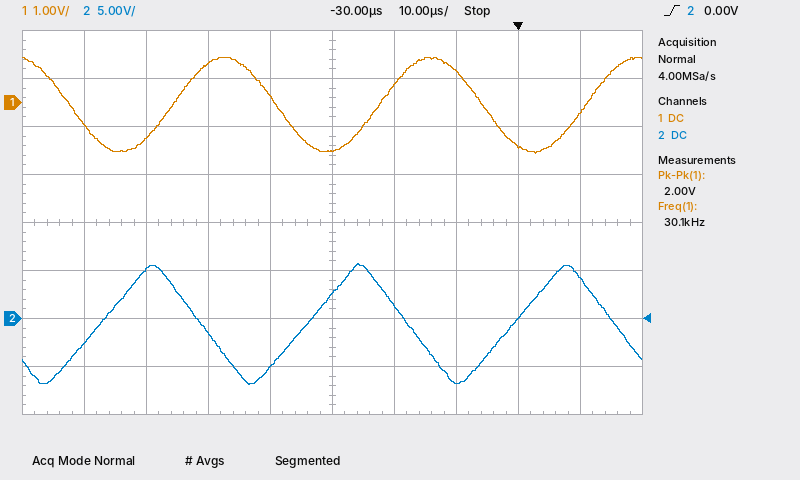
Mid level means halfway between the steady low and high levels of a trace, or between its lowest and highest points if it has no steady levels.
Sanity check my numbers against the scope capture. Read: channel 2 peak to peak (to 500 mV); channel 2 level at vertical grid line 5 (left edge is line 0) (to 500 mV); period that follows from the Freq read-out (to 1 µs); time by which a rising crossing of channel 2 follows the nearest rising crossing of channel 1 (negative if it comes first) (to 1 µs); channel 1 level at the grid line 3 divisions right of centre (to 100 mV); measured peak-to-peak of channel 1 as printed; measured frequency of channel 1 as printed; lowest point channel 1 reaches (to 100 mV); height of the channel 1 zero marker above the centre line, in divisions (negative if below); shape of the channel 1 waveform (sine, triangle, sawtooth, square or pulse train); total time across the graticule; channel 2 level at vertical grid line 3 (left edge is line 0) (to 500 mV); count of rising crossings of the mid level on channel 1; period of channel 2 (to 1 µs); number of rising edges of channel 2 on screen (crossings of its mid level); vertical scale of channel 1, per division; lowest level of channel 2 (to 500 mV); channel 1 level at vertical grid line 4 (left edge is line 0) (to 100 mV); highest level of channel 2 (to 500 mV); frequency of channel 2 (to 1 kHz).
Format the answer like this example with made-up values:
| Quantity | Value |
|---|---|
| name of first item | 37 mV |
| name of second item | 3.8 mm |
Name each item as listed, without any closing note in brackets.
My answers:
| Quantity | Value |
|---|---|
| channel 2 peak to peak | 12.5 V |
| channel 2 level at vertical grid line 5 (left edge is line 0) | 2.5 V |
| period that follows from the Freq read-out | 33 µs |
| time by which a rising crossing of channel 2 follows the nearest rising crossing of channel 1 (negative if it comes first) | -12 µs |
| channel 1 level at the grid line 3 divisions right of centre | -900 mV |
| measured peak-to-peak of channel 1 as printed | 2.00 V |
| measured frequency of channel 1 as printed | 30.1 kHz |
| lowest point channel 1 reaches | -1.1 V |
| height of the channel 1 zero marker above the centre line, in divisions | +2.5 div |
| shape of the channel 1 waveform | sine |
| total time across the graticule | 100 µs |
| channel 2 level at vertical grid line 3 (left edge is line 0) | -1.5 V |
| count of rising crossings of the mid level on channel 1 | 3 |
| period of channel 2 | 33 µs |
| number of rising edges of channel 2 on screen | 3 |
| vertical scale of channel 1, per division | 1 V |
| lowest level of channel 2 | -7.0 V |
| channel 1 level at vertical grid line 4 (left edge is line 0) | 100 mV |
| highest level of channel 2 | 5.5 V |
| frequency of channel 2 | 30 kHz |
